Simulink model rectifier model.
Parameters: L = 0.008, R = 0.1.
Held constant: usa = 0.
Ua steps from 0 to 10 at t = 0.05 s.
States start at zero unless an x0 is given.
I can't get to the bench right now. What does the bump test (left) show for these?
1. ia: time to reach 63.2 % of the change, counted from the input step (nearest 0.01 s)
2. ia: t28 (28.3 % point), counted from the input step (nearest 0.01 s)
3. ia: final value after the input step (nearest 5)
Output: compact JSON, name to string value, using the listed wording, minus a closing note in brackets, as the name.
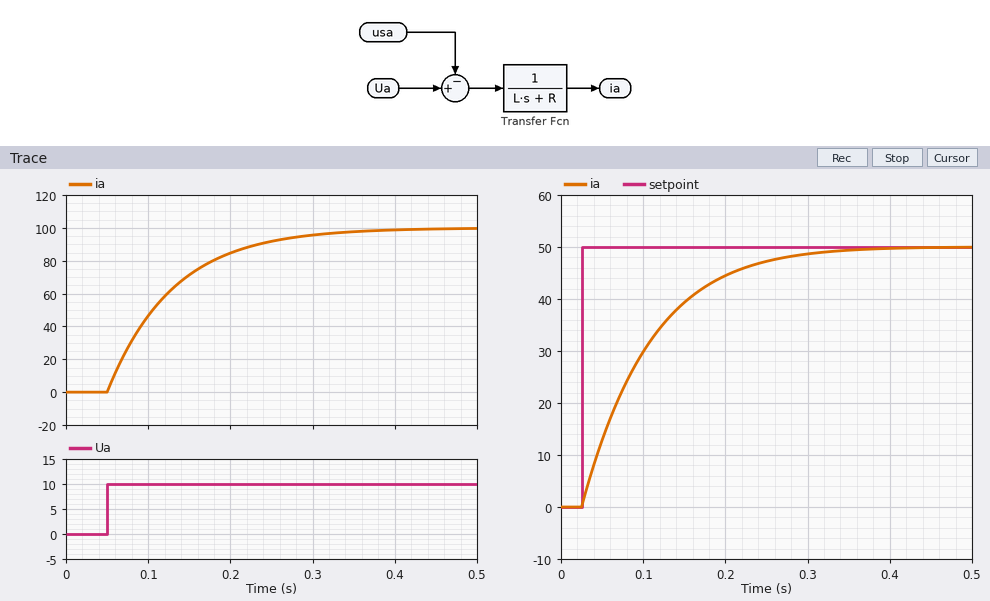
{"ia: time to reach 63.2 % of the change, counted from the input step": "0.08 s", "ia: t28 (28.3 % point), counted from the input step": "0.03 s", "ia: final value after the input step": "100"}
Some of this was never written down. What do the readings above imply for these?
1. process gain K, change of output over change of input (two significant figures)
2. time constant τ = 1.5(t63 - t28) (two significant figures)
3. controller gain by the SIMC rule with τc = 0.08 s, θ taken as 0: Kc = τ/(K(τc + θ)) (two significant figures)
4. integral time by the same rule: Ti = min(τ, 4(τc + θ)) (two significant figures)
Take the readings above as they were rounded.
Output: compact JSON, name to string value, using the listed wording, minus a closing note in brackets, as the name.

{"process gain K, change of output over change of input": "10", "time constant τ = 1.5(t63 - t28)": "0.075 s", "controller gain by the SIMC rule with τc = 0.08 s, θ taken as 0: Kc = τ/(K(τc + θ))": "0.094", "integral time by the same rule: Ti = min(τ, 4(τc + θ))": "0.075 s"}
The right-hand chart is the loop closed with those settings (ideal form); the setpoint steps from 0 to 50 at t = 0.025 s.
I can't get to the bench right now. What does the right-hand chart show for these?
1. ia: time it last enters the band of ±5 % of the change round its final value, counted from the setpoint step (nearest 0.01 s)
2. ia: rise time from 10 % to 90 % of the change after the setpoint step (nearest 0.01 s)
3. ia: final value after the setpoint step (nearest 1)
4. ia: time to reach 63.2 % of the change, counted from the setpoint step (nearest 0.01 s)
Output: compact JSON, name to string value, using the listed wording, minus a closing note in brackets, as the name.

{"ia: time it last enters the band of ±5 % of the change round its final value, counted from the setpoint step": "0.23 s", "ia: rise time from 10 % to 90 % of the change after the setpoint step": "0.17 s", "ia: final value after the setpoint step": "50", "ia: time to reach 63.2 % of the change, counted from the setpoint step": "0.08 s"}
